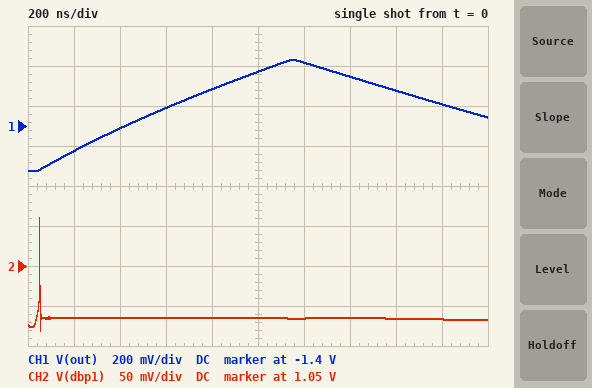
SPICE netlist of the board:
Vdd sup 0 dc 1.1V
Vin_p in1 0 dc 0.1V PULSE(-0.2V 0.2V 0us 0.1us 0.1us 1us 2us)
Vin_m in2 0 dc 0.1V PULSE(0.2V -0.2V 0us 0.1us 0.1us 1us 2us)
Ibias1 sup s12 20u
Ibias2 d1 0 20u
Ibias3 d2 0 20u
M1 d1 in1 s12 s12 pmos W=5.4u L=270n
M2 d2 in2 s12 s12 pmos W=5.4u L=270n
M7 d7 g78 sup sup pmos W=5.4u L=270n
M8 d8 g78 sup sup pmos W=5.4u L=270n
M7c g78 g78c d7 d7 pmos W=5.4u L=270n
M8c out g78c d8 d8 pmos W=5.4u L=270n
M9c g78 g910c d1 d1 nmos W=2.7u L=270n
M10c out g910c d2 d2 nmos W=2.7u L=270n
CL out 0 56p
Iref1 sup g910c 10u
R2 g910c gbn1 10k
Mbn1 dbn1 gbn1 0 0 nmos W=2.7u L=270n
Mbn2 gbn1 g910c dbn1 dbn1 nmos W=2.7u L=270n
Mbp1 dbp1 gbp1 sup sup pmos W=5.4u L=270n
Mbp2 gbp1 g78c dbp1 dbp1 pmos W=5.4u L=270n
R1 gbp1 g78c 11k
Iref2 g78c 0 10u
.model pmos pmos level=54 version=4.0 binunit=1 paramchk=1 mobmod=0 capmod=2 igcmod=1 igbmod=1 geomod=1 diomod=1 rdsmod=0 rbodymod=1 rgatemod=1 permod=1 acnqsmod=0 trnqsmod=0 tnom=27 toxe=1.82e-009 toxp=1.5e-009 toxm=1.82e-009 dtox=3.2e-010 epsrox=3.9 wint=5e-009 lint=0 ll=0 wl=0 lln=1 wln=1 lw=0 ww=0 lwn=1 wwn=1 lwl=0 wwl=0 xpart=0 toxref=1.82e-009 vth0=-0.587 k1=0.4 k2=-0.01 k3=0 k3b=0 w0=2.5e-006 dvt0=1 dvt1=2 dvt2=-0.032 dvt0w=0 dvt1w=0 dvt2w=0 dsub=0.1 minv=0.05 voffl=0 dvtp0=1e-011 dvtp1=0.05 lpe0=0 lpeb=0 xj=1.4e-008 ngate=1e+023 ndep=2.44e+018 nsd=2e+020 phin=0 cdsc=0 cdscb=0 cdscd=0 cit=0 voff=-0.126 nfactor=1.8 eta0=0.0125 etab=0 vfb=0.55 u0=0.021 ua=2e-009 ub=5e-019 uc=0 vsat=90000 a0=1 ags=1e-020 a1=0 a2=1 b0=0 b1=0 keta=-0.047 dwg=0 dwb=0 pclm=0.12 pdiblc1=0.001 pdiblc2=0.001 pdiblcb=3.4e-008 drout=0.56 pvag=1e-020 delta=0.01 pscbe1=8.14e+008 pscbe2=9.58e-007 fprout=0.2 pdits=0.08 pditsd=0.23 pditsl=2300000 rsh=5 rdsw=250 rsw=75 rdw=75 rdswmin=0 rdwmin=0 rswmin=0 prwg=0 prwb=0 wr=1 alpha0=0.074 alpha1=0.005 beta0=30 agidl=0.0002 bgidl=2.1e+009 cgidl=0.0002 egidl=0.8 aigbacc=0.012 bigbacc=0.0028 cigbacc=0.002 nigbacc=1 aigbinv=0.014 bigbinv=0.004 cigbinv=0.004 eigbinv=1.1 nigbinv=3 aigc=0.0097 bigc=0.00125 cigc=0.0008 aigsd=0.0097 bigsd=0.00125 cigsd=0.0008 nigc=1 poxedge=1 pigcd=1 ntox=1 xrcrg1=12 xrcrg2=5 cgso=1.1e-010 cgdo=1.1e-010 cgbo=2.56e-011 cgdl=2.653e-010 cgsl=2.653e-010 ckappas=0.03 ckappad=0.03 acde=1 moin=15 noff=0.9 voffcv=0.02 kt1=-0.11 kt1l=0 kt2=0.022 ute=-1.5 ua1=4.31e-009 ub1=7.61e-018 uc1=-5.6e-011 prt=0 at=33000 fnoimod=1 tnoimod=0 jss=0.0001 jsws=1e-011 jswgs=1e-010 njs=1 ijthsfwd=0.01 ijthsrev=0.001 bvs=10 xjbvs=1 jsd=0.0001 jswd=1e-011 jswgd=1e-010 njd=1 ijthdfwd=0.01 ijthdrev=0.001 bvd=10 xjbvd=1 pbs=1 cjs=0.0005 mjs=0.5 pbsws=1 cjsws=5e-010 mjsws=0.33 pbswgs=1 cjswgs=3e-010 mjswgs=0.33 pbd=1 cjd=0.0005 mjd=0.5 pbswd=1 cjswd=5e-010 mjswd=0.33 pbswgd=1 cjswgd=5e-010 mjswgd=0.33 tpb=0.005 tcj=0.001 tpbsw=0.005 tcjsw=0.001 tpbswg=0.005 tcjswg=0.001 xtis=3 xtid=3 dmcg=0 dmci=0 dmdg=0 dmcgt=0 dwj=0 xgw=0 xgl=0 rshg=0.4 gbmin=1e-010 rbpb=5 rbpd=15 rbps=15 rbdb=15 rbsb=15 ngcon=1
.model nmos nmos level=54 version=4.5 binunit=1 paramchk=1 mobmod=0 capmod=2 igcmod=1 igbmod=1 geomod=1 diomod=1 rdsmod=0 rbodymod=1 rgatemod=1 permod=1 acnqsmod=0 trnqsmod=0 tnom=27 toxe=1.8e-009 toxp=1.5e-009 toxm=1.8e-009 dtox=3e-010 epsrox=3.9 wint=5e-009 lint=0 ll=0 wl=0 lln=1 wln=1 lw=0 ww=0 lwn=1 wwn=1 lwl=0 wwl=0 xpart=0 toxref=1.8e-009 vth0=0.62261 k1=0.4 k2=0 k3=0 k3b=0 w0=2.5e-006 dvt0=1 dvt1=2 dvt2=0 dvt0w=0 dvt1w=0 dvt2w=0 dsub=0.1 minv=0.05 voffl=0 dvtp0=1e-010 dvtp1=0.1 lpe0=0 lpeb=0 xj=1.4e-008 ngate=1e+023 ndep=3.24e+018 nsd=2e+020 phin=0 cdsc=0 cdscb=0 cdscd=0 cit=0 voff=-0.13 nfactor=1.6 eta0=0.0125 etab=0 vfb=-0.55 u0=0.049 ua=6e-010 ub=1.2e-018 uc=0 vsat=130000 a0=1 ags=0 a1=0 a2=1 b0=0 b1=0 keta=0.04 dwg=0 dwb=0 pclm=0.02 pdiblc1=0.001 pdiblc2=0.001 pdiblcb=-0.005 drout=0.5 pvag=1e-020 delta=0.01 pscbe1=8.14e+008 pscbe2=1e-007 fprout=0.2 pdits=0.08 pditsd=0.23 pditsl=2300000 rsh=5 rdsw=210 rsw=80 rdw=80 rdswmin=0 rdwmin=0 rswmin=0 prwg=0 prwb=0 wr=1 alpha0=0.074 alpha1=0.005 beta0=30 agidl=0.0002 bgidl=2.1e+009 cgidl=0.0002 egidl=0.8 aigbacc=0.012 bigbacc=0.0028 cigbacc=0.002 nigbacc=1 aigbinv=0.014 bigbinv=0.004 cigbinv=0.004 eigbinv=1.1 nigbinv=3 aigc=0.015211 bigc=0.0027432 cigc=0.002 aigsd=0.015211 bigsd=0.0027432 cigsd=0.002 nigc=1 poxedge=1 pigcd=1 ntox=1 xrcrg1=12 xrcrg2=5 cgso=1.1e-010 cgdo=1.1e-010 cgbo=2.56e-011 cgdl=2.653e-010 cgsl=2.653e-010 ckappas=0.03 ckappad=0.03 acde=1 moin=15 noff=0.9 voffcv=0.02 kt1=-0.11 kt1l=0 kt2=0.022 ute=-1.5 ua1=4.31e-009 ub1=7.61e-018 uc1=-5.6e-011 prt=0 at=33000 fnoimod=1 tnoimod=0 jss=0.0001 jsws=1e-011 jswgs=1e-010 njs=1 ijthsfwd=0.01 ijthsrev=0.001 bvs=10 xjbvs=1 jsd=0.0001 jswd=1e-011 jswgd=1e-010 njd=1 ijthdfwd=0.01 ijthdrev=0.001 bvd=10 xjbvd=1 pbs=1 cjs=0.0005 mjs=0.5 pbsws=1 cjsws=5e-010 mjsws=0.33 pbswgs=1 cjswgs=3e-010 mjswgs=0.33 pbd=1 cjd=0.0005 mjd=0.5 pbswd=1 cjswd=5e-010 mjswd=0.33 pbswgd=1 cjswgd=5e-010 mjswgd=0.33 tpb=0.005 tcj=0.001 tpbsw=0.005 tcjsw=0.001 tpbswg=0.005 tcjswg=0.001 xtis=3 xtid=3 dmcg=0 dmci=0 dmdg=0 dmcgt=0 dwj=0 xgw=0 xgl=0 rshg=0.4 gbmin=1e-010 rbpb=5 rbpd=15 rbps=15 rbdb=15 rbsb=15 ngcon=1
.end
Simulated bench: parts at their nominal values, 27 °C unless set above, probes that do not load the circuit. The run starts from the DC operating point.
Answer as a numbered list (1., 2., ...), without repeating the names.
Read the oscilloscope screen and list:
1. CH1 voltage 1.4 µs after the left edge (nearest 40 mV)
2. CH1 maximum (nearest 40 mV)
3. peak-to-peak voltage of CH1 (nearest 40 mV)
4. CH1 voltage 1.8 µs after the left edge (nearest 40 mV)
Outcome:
1. -1.16 V
2. -1.08 V
3. 560 mV
4. -1.28 V
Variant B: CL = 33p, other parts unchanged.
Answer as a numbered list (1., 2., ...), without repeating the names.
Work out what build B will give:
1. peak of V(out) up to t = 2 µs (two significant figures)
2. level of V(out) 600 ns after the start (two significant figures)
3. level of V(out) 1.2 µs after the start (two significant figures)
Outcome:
1. -770 mV
2. -1.1 V
3. -790 mV
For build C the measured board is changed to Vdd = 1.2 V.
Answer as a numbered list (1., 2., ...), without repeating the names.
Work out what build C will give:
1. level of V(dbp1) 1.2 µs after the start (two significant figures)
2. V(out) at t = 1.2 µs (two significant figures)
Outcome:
1. 1.1 V
2. -1.0 V
